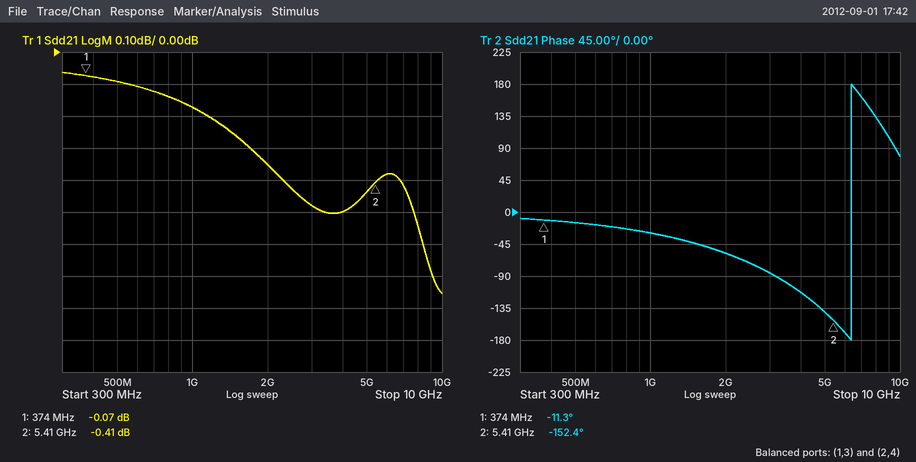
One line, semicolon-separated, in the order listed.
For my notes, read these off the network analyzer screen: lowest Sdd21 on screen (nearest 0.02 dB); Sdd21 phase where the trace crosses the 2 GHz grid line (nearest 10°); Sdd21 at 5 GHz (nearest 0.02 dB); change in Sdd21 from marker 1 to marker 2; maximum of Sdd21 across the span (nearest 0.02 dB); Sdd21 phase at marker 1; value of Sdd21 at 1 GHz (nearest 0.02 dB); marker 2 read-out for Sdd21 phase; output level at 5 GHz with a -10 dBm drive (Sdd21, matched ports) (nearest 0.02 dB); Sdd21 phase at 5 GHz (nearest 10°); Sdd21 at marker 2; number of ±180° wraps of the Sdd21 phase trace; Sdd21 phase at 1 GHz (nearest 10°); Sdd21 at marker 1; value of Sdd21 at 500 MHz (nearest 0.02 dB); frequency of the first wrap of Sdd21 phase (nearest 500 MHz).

-0.76 dB; -60°; -0.44 dB; -0.34 dB; -0.06 dB; -11.3°; -0.18 dB; -152.4°; -10.44 dBm; -140°; -0.41 dB; 1; -30°; -0.07 dB; -0.10 dB; 6.5 GHz
